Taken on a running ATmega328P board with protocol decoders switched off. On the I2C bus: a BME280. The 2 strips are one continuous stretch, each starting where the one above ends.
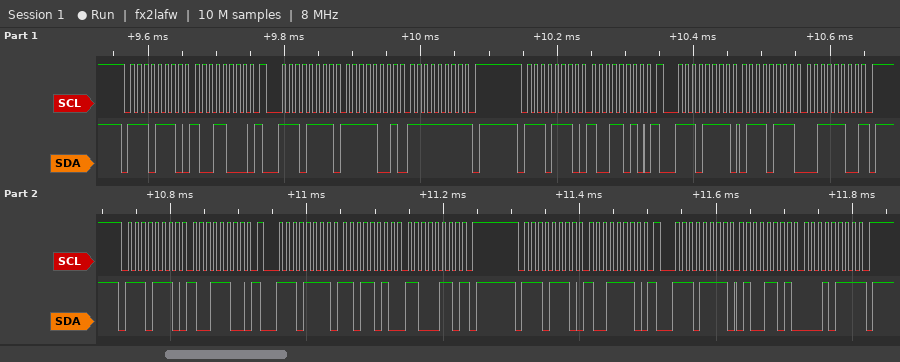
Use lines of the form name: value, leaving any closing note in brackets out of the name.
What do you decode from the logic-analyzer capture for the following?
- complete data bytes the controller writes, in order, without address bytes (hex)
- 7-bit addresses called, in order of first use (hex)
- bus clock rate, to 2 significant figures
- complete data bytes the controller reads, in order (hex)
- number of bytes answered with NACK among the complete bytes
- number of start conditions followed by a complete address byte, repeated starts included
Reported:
complete data bytes the controller writes, in order, without address bytes: 98 9A 9C 9E
7-bit addresses called, in order of first use: 0x77
bus clock rate, to 2 significant figures: 100 kHz
complete data bytes the controller reads, in order: F9 FF 77 3C DA C6 4D 17
number of bytes answered with NACK among the complete bytes: 4
number of start conditions followed by a complete address byte, repeated starts included: 8
